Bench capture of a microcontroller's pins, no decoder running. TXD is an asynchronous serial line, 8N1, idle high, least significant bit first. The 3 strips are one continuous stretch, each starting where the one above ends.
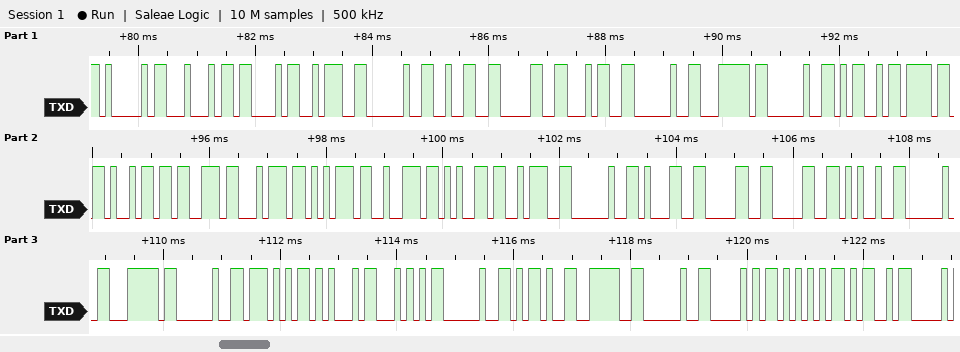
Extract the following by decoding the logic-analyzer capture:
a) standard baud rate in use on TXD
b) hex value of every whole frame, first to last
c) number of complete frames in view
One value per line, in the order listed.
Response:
9600 baud
41 44 43 3A 20 32 30 34 20 7C 20 4D 6F 69 73 74 75 72 65 3A 20 31 30 30 25 20 7C 20 57 45 54 20 2D 3E 20 50 55 4D
38
